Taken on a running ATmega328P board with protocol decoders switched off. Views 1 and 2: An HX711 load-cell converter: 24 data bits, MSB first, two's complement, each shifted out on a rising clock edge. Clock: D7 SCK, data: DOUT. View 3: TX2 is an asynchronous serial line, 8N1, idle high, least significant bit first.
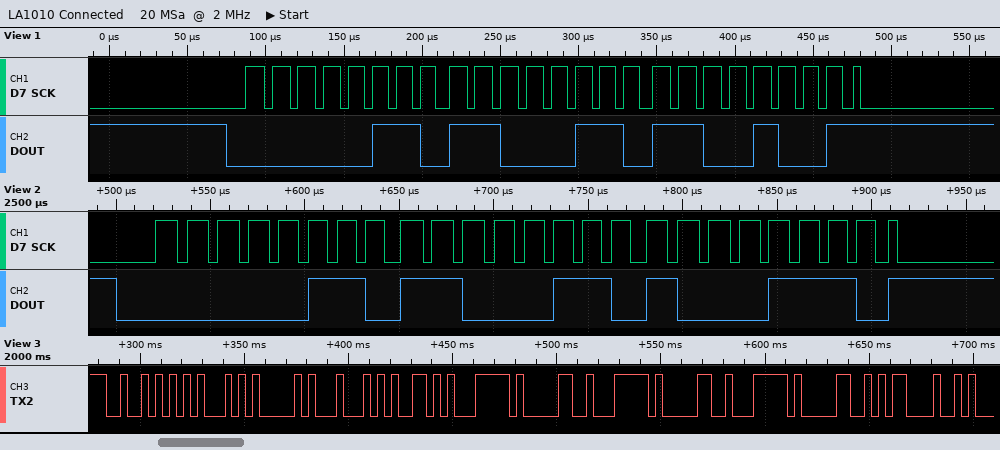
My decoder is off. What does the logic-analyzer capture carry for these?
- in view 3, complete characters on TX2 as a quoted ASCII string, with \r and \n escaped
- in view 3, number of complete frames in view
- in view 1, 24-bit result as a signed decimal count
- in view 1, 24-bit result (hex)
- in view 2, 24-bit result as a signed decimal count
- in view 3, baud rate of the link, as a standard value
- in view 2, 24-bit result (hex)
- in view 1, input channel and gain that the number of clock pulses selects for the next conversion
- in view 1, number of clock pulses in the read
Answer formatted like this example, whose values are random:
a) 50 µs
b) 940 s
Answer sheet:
a) "READY|0|0|0\r"
b) 12
c) 444105
d) 0x06C6C9
e) 444046
f) 300 baud
g) 0x06C68E
h) channel A, gain 128
i) 25
